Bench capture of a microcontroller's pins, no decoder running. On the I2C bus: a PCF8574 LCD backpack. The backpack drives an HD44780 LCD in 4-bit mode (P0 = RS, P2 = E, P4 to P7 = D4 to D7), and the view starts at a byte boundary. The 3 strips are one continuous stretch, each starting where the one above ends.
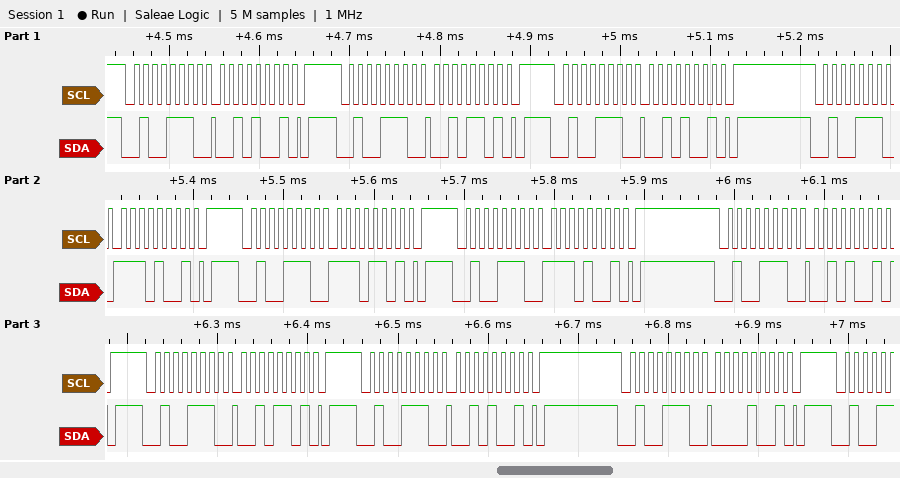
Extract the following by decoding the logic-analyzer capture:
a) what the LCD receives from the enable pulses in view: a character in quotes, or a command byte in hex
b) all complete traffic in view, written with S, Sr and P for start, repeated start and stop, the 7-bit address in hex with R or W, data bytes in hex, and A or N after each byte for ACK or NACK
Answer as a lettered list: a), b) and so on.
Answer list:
a) '.'
b) S 27W A 29 A P S 27W A 2D A P S 27W A 29 A P S 27W A E9 A P S 27W A ED A P S 27W A E9 A P S 27W A 29 A P S 27W A 2D A P S 27W A 29 A P S 27W A 09 A P
